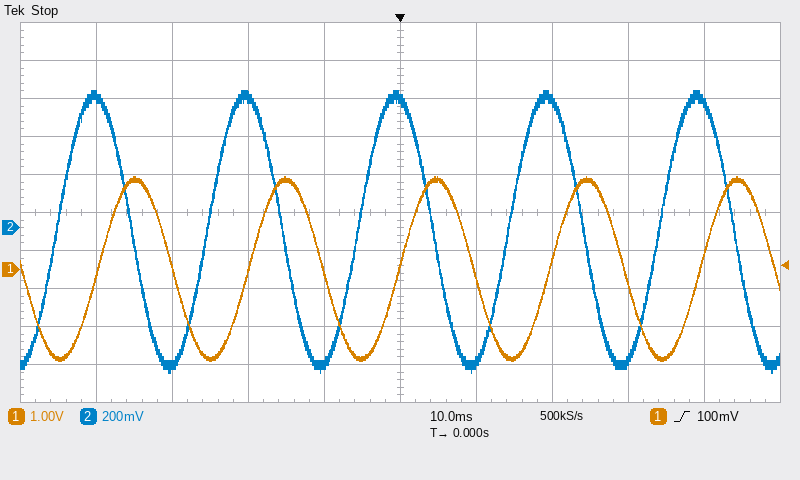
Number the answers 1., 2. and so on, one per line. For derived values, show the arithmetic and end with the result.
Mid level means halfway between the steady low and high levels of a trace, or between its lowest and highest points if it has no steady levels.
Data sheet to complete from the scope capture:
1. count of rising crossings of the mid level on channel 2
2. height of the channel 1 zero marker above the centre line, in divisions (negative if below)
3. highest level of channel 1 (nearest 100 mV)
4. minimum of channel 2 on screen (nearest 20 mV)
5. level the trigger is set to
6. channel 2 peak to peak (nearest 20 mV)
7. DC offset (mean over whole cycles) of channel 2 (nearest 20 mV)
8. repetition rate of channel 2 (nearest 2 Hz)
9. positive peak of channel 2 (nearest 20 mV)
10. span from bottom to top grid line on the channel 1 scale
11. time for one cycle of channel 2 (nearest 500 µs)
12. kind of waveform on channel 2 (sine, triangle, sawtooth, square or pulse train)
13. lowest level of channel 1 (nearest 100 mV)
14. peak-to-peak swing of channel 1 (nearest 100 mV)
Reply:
1. 5
2. -1.5 div
3. 2.4 V
4. -760 mV
5. 100 mV
6. 720 mV − (-760 mV) = 1.48 V
7. (720 mV + (-760 mV)) / 2 ≈ -20 mV
8. 1 / 20.0 ms ≈ 50 Hz
9. 720 mV
10. 10 V
11. 20.0 ms
12. sine
13. -2.4 V
14. 2.4 V − (-2.4 V) = 4.8 V
